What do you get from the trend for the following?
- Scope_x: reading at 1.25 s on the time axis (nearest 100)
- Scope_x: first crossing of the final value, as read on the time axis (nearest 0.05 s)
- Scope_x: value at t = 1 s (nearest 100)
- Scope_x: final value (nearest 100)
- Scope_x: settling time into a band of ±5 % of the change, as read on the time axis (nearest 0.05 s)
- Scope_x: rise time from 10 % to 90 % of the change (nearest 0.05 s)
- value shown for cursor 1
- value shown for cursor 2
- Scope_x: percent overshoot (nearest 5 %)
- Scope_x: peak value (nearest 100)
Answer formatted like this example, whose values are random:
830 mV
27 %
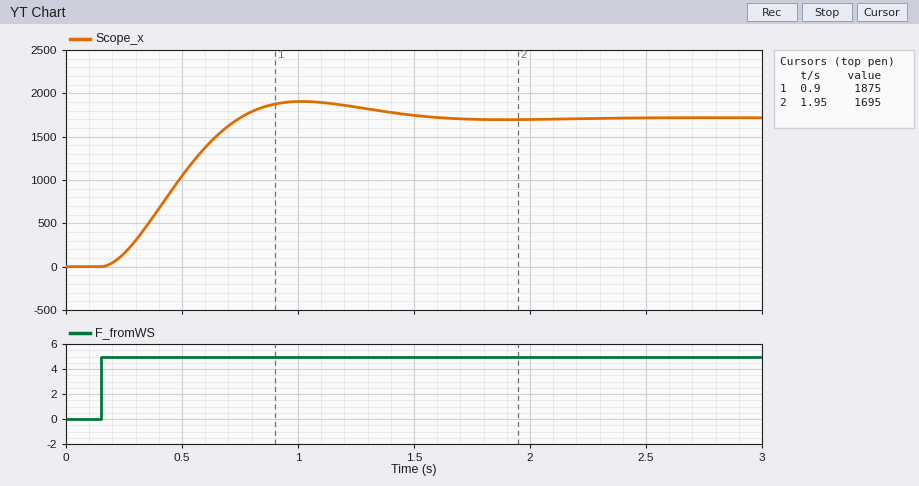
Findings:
1800
0.75 s
1900
1700
1.35 s
0.40 s
1875
1695
10 %
1900
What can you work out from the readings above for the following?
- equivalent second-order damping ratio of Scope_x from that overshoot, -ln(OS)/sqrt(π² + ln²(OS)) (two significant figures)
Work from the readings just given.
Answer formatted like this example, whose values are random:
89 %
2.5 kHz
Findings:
0.59
